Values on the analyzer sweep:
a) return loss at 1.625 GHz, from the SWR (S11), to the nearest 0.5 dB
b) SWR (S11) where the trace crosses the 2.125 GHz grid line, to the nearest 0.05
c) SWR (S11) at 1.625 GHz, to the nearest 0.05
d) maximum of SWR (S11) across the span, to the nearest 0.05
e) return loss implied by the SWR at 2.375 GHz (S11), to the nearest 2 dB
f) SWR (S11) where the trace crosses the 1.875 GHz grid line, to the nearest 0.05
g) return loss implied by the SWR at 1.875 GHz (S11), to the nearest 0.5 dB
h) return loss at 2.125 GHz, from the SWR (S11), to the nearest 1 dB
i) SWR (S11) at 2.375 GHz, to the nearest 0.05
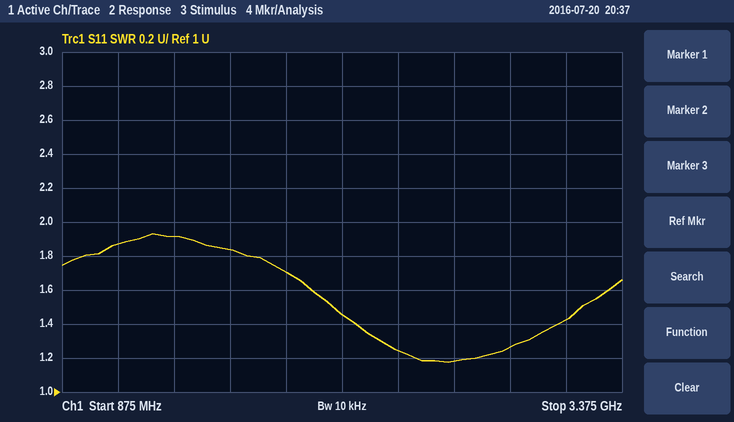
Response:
10.5 dB
1.45
1.85
1.95
20 dB
1.70
11.5 dB
15 dB
1.25
